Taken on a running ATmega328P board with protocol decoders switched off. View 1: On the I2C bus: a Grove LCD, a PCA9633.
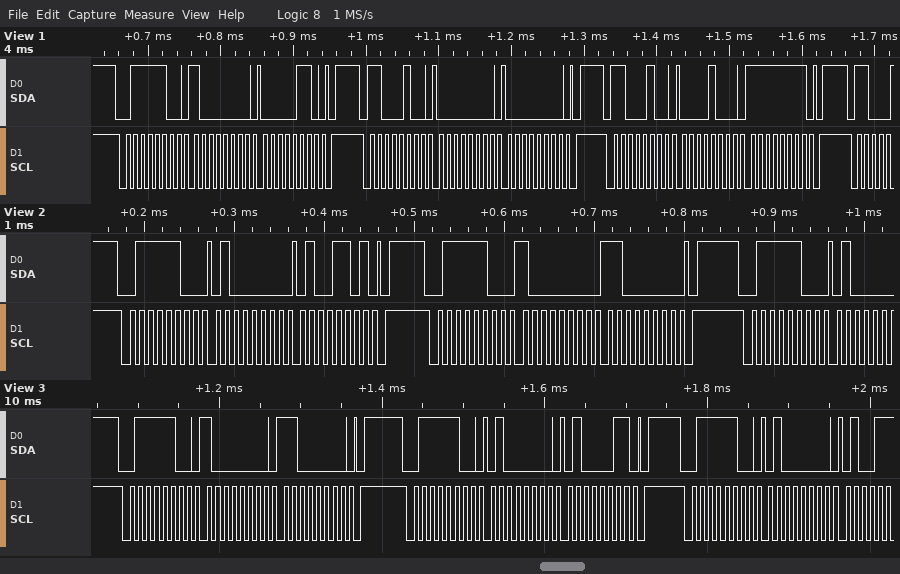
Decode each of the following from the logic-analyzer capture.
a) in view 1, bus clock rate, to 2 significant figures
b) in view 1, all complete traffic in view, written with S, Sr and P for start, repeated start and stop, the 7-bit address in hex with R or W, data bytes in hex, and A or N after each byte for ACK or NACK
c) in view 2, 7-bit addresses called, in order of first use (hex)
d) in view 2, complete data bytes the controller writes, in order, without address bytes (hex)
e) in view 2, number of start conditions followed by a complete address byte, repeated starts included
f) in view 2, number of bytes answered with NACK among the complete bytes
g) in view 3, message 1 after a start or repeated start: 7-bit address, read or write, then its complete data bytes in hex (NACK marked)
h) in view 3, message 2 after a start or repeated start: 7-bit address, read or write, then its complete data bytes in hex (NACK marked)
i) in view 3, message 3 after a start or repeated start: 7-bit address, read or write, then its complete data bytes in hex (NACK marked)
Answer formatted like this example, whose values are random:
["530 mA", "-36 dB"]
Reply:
["100 kHz", "S 3EW A 80 A 06 A P S 62W A 00 A 00 A P S 62W A 08 A FF A P", "0x3E", "40 4D 80 C0", "3", "0", "0x3E write: 80 C0", "0x3E write: 40 43", "0x3E write: 40"]
